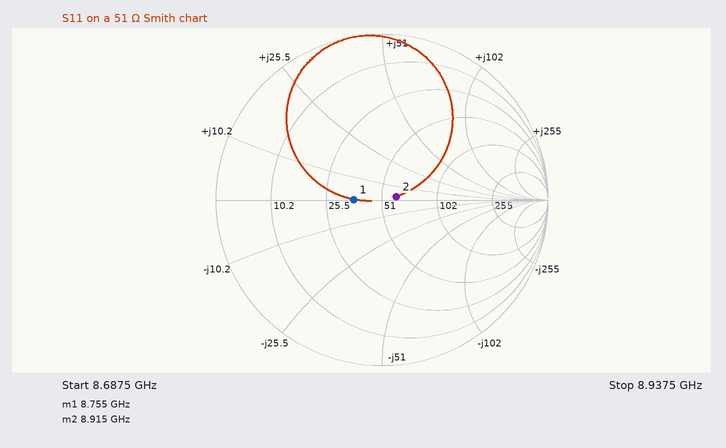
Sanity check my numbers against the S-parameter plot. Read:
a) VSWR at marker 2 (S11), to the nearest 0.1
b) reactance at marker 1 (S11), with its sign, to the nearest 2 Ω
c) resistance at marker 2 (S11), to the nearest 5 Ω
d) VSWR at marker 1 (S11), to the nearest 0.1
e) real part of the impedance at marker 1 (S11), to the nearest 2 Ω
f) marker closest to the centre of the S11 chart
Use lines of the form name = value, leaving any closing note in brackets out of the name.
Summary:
VSWR at marker 2 (S11), to the nearest 0.1 = 1.2
reactance at marker 1 (S11), with its sign, to the nearest 2 Ω = 0 Ω
resistance at marker 2 (S11), to the nearest 5 Ω = 60 Ω
VSWR at marker 1 (S11), to the nearest 0.1 = 1.4
real part of the impedance at marker 1 (S11), to the nearest 2 Ω = 36 Ω
marker closest to the centre of the S11 chart = marker 2
